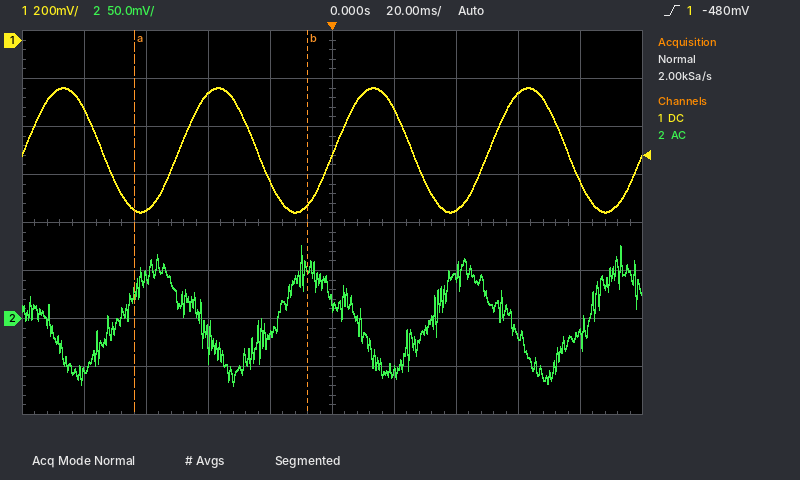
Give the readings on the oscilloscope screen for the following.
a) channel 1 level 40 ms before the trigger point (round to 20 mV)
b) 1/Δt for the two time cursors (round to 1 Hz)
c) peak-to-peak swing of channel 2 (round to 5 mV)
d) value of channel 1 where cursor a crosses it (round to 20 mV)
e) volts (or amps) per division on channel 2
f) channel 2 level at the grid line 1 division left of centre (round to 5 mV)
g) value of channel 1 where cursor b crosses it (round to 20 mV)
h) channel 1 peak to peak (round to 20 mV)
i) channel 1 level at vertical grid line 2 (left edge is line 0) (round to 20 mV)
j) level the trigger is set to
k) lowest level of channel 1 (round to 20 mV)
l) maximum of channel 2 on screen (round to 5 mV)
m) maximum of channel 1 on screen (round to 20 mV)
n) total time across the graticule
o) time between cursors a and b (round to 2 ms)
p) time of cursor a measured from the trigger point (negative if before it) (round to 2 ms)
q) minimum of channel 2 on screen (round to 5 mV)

-220 mV
18 Hz
145 mV
-700 mV
50 mV
-15 mV
-680 mV
520 mV
-700 mV
-480 mV
-720 mV
75 mV
-200 mV
200 ms
56 ms
-64 ms
-70 mV
